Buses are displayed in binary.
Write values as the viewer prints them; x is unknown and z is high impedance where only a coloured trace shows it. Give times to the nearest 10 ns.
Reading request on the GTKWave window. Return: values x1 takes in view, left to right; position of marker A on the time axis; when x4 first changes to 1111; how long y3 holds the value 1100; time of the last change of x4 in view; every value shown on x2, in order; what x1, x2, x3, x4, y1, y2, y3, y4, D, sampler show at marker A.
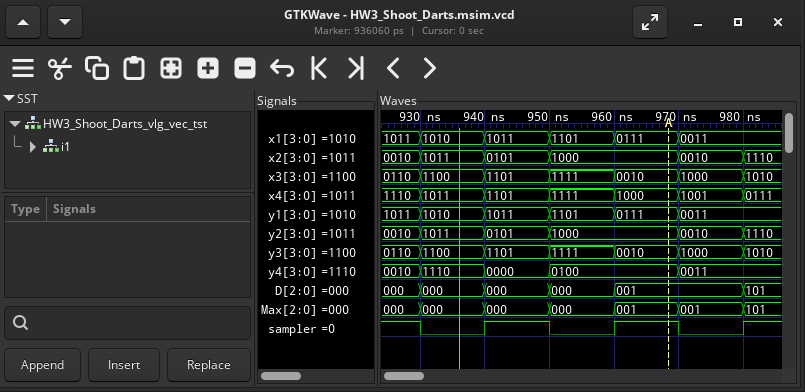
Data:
1011, 1010, 1011, 1101, 0111, 0011
970 ns
950 ns
10 ns
980 ns
0010, 1011, 0101, 1000, 0010, 1110
x1=0111, x2=1000, x3=0010, x4=1000, y1=0111, y2=1000, y3=0010, y4=0100, D=001, sampler=1
